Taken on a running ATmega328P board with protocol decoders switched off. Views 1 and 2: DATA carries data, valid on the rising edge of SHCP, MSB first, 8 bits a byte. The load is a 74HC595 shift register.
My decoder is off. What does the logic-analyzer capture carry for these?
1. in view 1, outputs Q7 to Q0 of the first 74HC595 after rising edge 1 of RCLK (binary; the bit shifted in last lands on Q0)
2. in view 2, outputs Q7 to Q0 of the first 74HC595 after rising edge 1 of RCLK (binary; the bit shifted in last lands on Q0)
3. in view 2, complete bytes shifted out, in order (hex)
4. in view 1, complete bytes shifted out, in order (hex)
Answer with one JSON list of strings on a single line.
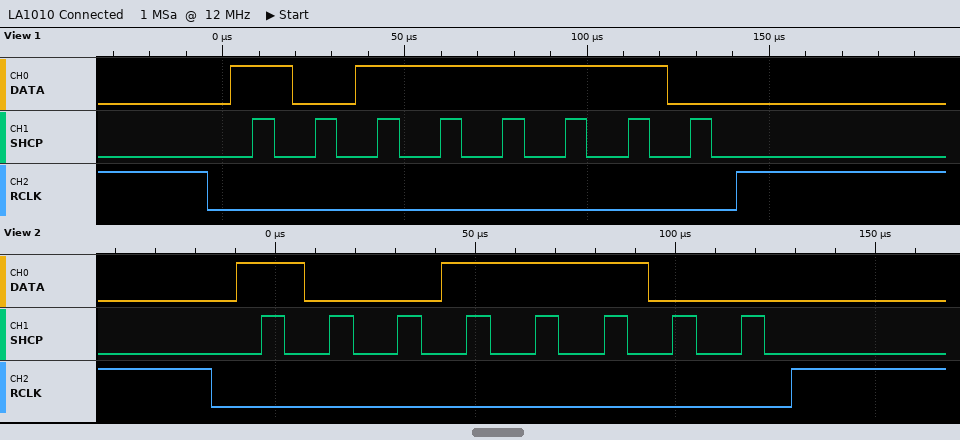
["10111110", "10011100", "0x9C", "BE"]
